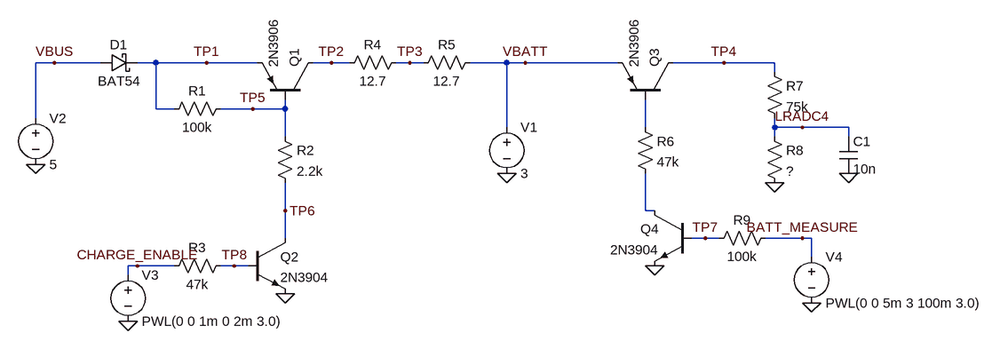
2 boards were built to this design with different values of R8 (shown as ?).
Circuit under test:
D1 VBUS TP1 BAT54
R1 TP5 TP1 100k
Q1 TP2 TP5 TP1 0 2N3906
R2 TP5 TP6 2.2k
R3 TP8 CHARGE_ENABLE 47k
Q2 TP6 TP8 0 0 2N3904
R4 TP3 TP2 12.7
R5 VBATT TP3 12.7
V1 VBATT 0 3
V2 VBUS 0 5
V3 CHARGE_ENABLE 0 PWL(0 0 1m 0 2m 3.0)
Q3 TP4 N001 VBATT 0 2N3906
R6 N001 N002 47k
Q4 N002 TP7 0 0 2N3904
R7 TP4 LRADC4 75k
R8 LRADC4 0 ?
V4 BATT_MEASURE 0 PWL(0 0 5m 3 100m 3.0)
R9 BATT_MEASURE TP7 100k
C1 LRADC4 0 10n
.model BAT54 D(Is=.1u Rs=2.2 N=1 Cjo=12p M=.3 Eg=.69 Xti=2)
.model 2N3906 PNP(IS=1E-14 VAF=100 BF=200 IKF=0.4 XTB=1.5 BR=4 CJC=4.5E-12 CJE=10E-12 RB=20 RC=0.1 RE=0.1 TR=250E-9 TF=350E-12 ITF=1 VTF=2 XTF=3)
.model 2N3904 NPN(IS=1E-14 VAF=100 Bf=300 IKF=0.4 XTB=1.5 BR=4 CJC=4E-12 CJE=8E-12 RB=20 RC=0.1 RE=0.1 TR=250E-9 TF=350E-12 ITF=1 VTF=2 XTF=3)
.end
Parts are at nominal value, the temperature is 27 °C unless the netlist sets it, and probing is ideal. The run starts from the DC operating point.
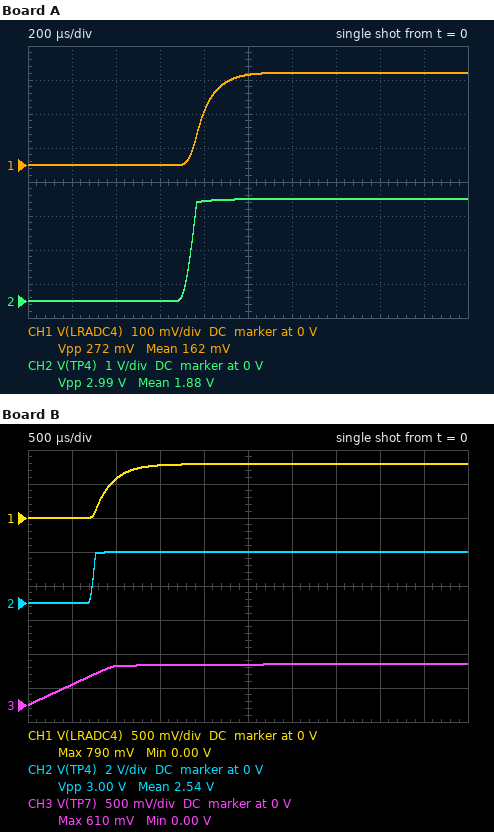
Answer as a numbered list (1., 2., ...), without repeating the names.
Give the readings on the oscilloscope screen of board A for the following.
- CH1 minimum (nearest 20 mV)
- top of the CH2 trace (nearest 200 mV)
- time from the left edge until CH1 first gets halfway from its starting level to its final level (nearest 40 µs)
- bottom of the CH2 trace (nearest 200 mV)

1. 0 V
2. 3.0 V
3. 800 µs
4. 0 V
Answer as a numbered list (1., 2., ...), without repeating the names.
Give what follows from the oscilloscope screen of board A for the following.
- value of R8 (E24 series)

1. 7.5 kΩ
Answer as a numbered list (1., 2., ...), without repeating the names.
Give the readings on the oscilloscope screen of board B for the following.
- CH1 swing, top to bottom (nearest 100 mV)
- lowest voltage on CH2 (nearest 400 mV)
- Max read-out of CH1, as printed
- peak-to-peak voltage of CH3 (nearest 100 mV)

1. 800 mV
2. 0 V
3. 790 mV
4. 600 mV
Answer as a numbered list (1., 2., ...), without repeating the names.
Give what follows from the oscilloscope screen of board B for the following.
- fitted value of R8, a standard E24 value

1. 27 kΩ
